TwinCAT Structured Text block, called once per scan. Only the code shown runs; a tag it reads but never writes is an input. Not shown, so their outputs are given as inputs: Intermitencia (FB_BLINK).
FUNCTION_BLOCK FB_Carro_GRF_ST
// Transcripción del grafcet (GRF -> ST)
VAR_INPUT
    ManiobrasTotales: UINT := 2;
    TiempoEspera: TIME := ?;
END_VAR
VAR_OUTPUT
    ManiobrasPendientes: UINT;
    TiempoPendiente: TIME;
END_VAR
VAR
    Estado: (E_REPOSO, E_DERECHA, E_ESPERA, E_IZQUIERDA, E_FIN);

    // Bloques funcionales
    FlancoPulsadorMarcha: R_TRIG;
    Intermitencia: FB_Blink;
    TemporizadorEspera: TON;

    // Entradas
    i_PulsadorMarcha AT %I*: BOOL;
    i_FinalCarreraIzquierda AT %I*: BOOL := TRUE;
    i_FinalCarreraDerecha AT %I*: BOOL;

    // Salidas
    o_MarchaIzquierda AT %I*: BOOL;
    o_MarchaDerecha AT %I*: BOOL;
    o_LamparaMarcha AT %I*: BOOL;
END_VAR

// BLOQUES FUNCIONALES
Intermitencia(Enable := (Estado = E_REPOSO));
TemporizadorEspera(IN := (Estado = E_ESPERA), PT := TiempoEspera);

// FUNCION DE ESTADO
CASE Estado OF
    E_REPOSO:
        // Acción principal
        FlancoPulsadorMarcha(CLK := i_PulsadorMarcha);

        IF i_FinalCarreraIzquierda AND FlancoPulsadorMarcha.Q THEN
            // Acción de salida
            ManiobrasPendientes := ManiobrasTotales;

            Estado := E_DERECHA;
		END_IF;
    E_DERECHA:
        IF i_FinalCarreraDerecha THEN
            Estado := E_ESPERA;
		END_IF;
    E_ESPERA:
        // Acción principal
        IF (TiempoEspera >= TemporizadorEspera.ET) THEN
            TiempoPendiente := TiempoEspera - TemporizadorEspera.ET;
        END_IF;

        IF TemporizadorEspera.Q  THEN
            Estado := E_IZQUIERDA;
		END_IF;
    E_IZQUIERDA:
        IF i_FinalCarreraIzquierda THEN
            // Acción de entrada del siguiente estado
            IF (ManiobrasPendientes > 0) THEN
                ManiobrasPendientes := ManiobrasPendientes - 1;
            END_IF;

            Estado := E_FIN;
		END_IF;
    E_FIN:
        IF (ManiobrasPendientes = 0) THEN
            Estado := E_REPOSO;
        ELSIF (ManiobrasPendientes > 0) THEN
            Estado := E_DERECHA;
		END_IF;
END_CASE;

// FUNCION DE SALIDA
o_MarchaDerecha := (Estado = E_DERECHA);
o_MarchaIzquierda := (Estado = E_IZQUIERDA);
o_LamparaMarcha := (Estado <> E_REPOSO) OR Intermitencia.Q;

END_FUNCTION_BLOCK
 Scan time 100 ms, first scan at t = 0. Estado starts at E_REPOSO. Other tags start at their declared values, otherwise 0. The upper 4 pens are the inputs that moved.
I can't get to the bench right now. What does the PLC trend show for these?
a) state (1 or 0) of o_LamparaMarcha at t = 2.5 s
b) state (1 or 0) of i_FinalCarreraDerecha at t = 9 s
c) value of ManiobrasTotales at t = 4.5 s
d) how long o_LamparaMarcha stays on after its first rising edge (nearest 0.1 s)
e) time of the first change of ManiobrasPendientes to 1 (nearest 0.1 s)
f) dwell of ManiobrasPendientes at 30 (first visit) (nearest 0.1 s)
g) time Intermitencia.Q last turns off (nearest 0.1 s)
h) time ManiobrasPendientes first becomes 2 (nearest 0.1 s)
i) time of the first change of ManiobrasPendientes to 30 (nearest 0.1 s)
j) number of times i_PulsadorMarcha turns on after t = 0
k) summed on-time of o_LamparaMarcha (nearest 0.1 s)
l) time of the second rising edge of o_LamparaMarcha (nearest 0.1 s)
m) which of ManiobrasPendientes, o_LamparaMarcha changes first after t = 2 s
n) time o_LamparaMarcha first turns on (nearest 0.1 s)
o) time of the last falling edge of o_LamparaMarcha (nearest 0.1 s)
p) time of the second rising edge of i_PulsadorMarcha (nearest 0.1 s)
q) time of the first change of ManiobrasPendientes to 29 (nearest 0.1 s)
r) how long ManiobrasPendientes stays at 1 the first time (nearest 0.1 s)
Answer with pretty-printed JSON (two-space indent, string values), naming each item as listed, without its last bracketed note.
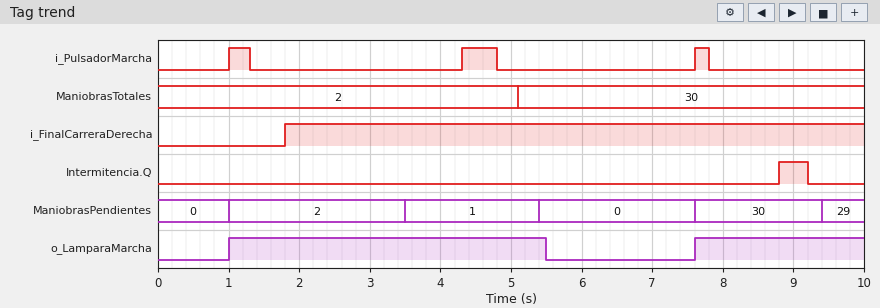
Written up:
{
  "state (1 or 0) of o_LamparaMarcha at t = 2.5 s": "1",
  "state (1 or 0) of i_FinalCarreraDerecha at t = 9 s": "1",
  "value of ManiobrasTotales at t = 4.5 s": "2",
  "how long o_LamparaMarcha stays on after its first rising edge": "4.5 s",
  "time of the first change of ManiobrasPendientes to 1": "3.5 s",
  "dwell of ManiobrasPendientes at 30 (first visit)": "1.8 s",
  "time Intermitencia.Q last turns off": "9.2 s",
  "time ManiobrasPendientes first becomes 2": "1.0 s",
  "time of the first change of ManiobrasPendientes to 30": "7.6 s",
  "number of times i_PulsadorMarcha turns on after t = 0": "3",
  "summed on-time of o_LamparaMarcha": "6.9 s",
  "time of the second rising edge of o_LamparaMarcha": "7.6 s",
  "which of ManiobrasPendientes, o_LamparaMarcha changes first after t = 2 s": "ManiobrasPendientes",
  "time o_LamparaMarcha first turns on": "1.0 s",
  "time of the last falling edge of o_LamparaMarcha": "5.5 s",
  "time of the second rising edge of i_PulsadorMarcha": "4.3 s",
  "time of the first change of ManiobrasPendientes to 29": "9.4 s",
  "how long ManiobrasPendientes stays at 1 the first time": "1.9 s"
}
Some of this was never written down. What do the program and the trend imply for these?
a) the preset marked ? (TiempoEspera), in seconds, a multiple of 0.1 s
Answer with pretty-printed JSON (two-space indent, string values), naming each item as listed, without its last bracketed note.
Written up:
{
  "the preset marked ? (TiempoEspera), in seconds, a multiple of 0.1 s": "1.5 s"
}
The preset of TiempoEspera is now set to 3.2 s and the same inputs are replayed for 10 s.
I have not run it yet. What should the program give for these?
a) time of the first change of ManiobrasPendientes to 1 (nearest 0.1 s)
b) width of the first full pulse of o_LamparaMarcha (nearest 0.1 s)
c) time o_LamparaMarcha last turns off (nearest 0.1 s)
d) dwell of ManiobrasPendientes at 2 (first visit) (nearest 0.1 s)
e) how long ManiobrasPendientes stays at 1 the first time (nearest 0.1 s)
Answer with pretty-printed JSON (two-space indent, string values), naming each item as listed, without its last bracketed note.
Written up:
{
  "time of the first change of ManiobrasPendientes to 1": "5.2 s",
  "width of the first full pulse of o_LamparaMarcha": "8.2 s",
  "time o_LamparaMarcha last turns off": "9.2 s",
  "dwell of ManiobrasPendientes at 2 (first visit)": "4.2 s",
  "how long ManiobrasPendientes stays at 1 the first time": "3.6 s"
}
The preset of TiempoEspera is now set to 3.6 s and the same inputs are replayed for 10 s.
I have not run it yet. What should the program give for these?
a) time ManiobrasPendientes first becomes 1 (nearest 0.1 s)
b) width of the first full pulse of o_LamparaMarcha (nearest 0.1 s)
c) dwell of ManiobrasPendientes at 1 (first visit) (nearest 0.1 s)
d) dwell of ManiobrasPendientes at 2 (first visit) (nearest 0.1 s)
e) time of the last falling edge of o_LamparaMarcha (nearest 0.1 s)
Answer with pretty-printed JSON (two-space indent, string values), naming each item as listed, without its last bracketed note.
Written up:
{
  "time ManiobrasPendientes first becomes 1": "5.6 s",
  "width of the first full pulse of o_LamparaMarcha": "8.7 s",
  "dwell of ManiobrasPendientes at 1 (first visit)": "4.0 s",
  "dwell of ManiobrasPendientes at 2 (first visit)": "4.6 s",
  "time of the last falling edge of o_LamparaMarcha": "9.7 s"
}
